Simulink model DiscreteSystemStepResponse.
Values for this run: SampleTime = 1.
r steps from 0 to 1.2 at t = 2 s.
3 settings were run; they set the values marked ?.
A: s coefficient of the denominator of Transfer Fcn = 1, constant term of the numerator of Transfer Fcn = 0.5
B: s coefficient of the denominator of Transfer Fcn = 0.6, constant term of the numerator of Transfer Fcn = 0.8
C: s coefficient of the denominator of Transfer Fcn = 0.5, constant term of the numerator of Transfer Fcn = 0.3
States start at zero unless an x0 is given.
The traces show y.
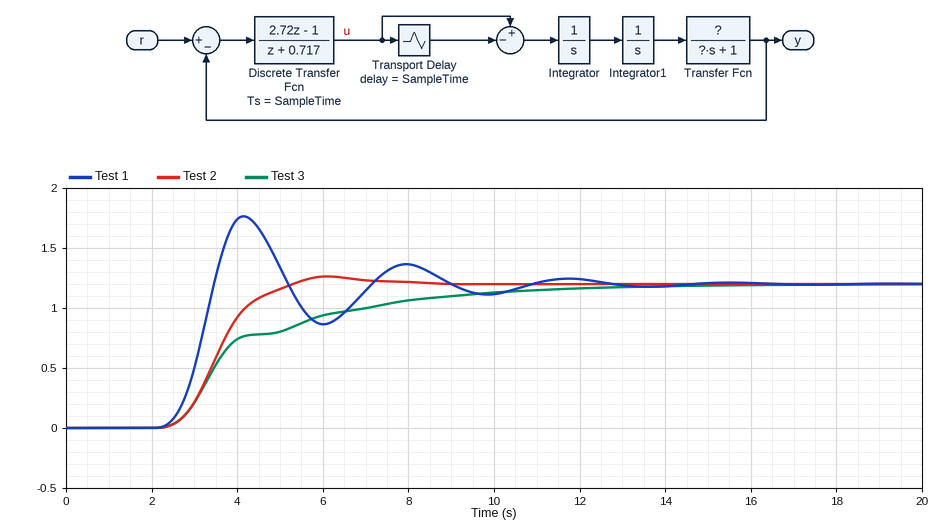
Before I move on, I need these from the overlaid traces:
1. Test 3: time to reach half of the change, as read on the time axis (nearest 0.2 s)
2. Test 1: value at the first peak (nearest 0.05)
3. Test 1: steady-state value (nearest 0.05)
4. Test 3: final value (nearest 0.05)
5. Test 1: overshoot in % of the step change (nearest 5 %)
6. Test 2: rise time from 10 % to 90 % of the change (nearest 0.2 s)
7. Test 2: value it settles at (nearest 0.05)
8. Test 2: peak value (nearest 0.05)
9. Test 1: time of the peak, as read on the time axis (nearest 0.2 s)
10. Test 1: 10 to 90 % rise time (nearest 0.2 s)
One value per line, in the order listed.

3.6 s
1.75
1.20
1.20
45 %
1.6 s
1.20
1.25
4.2 s
0.8 s
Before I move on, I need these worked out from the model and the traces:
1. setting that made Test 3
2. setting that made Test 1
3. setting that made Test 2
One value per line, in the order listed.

C
B
A
